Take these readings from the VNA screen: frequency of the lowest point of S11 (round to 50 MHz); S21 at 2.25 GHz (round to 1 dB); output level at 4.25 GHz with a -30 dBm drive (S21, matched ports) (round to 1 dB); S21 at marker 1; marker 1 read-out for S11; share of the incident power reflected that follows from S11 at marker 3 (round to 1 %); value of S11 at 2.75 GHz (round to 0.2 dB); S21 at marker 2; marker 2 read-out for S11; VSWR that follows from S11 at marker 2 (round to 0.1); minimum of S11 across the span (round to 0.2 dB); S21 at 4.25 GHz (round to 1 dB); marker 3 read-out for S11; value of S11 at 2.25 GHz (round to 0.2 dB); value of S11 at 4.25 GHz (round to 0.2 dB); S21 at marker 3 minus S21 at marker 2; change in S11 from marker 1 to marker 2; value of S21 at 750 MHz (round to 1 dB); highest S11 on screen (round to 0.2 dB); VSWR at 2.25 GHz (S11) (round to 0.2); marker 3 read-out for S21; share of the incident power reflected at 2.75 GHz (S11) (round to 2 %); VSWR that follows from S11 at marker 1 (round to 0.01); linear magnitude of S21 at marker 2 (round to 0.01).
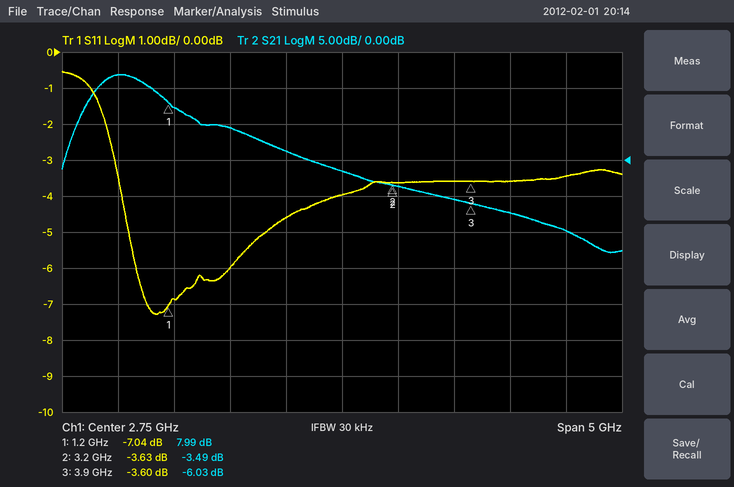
1.10 GHz
1 dB
-37 dBm
7.99 dB
-7.04 dB
44 %
-4.0 dB
-3.49 dB
-3.63 dB
4.9
-7.2 dB
-7 dB
-3.60 dB
-4.6 dB
-3.6 dB
-2.54 dB
3.41 dB
12 dB
-0.6 dB
3.8
-6.03 dB
40 %
2.60
0.67
